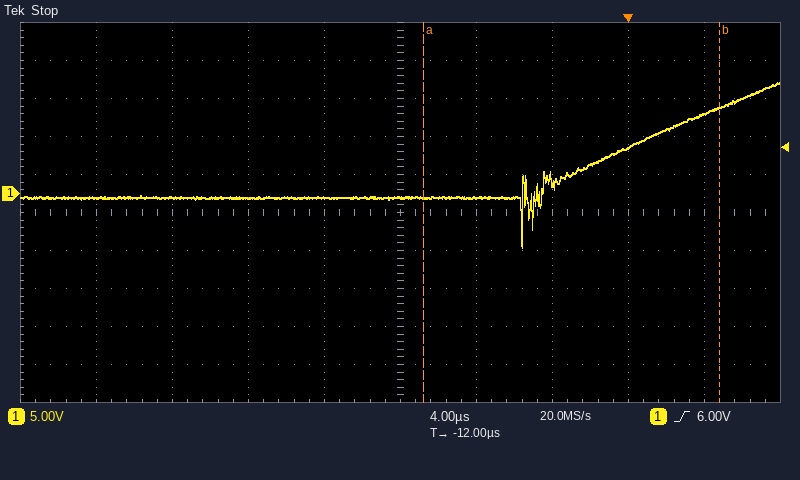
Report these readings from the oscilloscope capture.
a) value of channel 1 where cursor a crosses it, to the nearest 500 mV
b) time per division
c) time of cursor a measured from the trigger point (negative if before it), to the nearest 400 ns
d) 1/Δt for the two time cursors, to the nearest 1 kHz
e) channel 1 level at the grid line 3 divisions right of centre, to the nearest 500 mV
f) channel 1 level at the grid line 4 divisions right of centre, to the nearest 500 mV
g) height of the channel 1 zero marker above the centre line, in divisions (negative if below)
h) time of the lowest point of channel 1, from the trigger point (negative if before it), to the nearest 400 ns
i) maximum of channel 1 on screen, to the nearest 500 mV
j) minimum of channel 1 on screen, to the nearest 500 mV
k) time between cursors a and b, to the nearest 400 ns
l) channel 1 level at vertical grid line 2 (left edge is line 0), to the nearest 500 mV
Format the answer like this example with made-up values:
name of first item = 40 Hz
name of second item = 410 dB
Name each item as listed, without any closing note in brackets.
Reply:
value of channel 1 where cursor a crosses it, to the nearest 500 mV = -500 mV
time per division = 4 µs
time of cursor a measured from the trigger point (negative if before it), to the nearest 400 ns = -10.8 µs
1/Δt for the two time cursors, to the nearest 1 kHz = 64 kHz
channel 1 level at the grid line 3 divisions right of centre, to the nearest 500 mV = 6.0 V
channel 1 level at the grid line 4 divisions right of centre, to the nearest 500 mV = 10.5 V
height of the channel 1 zero marker above the centre line, in divisions = +0.5 div
time of the lowest point of channel 1, from the trigger point (negative if before it), to the nearest 400 ns = -5.6 µs
maximum of channel 1 on screen, to the nearest 500 mV = 14.5 V
minimum of channel 1 on screen, to the nearest 500 mV = -7.0 V
time between cursors a and b, to the nearest 400 ns = 15.6 µs
channel 1 level at vertical grid line 2 (left edge is line 0), to the nearest 500 mV = -500 mV
